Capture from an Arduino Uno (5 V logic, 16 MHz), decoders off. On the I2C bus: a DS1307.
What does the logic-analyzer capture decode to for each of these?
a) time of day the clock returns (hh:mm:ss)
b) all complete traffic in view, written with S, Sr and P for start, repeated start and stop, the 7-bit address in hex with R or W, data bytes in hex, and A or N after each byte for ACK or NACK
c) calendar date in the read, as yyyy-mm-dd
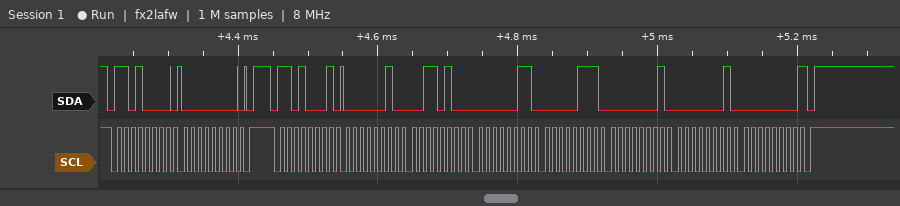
03:34:02
S 68W A 00 A P S 68R A 02 A 34 A 03 A 07 A 01 A 01 A 00 N P
2000-01-01
